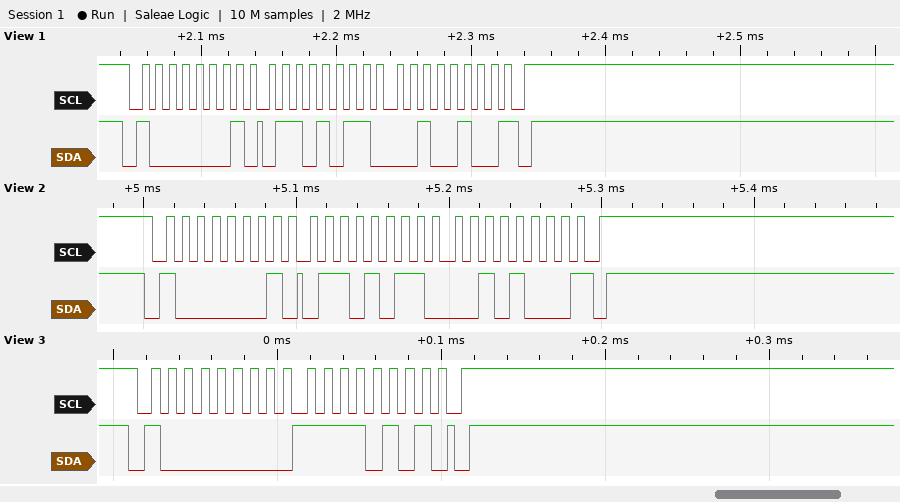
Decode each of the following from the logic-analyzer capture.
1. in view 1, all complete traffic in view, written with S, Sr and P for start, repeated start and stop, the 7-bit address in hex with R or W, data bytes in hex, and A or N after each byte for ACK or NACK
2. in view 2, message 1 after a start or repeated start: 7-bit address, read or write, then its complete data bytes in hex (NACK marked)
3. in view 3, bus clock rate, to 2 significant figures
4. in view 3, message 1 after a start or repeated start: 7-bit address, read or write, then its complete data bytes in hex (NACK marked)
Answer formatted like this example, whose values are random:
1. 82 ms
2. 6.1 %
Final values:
1. S 40R A 6B A 24 N P
2. 0x40 read: 6B 28 NACK
3. 100 kHz
4. 0x40 write: F5
